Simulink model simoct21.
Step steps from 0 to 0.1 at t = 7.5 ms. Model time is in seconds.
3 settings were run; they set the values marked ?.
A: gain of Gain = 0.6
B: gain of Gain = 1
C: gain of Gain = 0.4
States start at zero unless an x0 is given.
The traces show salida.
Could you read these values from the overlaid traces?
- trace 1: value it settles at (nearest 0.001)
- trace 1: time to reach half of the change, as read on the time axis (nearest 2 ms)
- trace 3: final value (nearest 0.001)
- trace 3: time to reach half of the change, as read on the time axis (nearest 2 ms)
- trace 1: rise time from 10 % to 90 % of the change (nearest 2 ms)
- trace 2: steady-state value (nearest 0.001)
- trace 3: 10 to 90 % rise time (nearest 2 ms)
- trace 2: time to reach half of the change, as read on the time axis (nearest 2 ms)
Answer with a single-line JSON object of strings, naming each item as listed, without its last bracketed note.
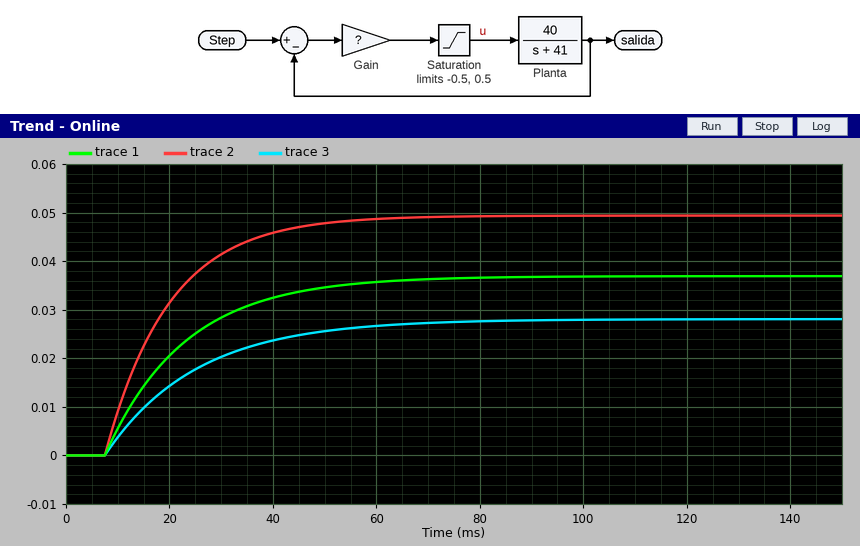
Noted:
{"trace 1: value it settles at": "0.037", "trace 1: time to reach half of the change, as read on the time axis": "18 ms", "trace 3: final value": "0.028", "trace 3: time to reach half of the change, as read on the time axis": "20 ms", "trace 1: rise time from 10 % to 90 % of the change": "34 ms", "trace 2: steady-state value": "0.049", "trace 3: 10 to 90 % rise time": "38 ms", "trace 2: time to reach half of the change, as read on the time axis": "16 ms"}
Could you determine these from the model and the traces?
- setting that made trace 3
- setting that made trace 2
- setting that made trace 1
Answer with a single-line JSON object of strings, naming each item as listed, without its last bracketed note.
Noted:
{"setting that made trace 3": "C", "setting that made trace 2": "B", "setting that made trace 1": "A"}
